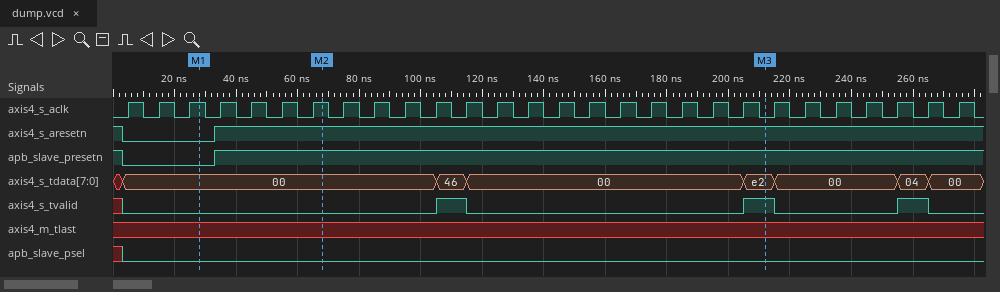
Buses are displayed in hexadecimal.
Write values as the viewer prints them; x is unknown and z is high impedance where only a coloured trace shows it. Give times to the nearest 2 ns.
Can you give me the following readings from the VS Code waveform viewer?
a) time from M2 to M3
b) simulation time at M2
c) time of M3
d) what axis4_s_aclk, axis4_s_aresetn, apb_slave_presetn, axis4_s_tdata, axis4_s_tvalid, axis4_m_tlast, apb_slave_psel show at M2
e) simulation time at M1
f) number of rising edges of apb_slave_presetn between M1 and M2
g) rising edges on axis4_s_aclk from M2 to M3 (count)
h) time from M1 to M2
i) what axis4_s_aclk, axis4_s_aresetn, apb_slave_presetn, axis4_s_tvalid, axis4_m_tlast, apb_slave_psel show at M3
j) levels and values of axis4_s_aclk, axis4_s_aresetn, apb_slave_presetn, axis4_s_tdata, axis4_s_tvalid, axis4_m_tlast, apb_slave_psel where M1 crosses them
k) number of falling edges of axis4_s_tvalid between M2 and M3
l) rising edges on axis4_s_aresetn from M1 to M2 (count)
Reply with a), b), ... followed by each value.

a) 144 ns
b) 68 ns
c) 212 ns
d) axis4_s_aclk=1, axis4_s_aresetn=1, apb_slave_presetn=1, axis4_s_tdata=00, axis4_s_tvalid=0, axis4_m_tlast=x, apb_slave_psel=0
e) 28 ns
f) 1
g) 14
h) 40 ns
i) axis4_s_aclk=0, axis4_s_aresetn=1, apb_slave_presetn=1, axis4_s_tvalid=1, axis4_m_tlast=x, apb_slave_psel=0
j) axis4_s_aclk=1, axis4_s_aresetn=0, apb_slave_presetn=0, axis4_s_tdata=00, axis4_s_tvalid=0, axis4_m_tlast=x, apb_slave_psel=0
k) 1
l) 1
